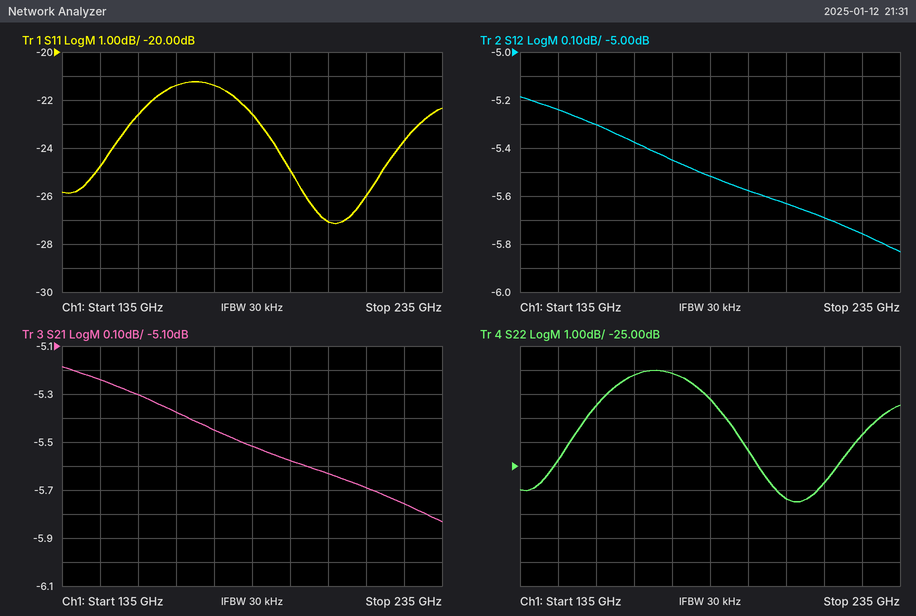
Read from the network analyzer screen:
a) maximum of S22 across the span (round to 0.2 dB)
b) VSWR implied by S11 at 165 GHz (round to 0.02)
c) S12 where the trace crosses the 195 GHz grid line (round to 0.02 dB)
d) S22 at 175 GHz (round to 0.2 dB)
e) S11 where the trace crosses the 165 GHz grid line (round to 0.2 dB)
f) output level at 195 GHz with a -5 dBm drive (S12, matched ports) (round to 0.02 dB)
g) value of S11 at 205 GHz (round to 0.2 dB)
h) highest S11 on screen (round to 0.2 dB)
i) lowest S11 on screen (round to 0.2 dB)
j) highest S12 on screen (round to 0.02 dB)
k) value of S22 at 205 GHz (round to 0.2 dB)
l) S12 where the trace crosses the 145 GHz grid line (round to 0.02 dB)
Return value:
-21.0 dB
1.18
-5.58 dB
-21.2 dB
-21.4 dB
-10.58 dBm
-27.0 dB
-21.2 dB
-27.2 dB
-5.18 dB
-26.4 dB
-5.24 dB
